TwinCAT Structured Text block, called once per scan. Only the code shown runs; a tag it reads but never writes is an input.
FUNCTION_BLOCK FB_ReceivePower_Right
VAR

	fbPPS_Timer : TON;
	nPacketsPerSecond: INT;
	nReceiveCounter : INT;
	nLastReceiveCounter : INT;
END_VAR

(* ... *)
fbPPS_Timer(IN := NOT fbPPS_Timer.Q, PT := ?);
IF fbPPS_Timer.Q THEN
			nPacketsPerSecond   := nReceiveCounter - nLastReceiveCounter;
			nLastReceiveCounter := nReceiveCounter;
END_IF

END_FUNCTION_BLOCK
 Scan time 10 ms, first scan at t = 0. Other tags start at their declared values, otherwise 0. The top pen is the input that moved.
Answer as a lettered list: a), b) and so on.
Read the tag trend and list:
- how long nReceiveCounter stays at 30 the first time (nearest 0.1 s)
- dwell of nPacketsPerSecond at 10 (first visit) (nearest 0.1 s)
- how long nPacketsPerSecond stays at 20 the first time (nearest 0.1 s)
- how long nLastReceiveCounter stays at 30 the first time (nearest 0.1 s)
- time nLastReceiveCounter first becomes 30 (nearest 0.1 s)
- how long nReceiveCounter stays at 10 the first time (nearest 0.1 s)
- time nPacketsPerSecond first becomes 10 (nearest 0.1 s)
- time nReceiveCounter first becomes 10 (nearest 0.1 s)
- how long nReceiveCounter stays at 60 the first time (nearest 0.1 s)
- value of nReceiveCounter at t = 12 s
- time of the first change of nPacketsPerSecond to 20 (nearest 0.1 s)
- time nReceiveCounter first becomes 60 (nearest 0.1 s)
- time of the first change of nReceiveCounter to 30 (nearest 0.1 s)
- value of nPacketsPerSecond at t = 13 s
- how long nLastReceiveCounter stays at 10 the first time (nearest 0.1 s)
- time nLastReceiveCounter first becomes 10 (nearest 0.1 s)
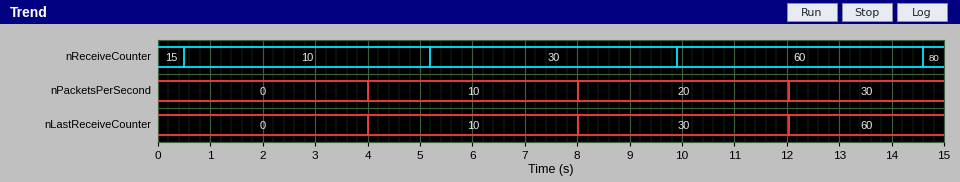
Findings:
a) 4.7 s
b) 4.0 s
c) 4.0 s
d) 4.0 s
e) 8.0 s
f) 4.7 s
g) 4.0 s
h) 0.5 s
i) 4.7 s
j) 60
k) 8.0 s
l) 9.9 s
m) 5.2 s
n) 30
o) 4.0 s
p) 4.0 s
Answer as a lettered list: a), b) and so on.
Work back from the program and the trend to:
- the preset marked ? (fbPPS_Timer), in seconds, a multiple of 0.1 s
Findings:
a) 4.0 s
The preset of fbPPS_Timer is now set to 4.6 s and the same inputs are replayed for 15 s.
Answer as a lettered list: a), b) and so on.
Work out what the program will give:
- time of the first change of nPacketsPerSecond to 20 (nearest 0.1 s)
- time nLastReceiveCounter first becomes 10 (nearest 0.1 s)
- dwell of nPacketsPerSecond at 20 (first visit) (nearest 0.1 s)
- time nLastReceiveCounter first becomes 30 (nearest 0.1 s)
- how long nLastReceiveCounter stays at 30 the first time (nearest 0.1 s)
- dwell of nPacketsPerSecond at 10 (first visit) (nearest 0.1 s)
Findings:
a) 9.2 s
b) 4.6 s
c) 4.6 s
d) 9.2 s
e) 4.6 s
f) 4.6 s
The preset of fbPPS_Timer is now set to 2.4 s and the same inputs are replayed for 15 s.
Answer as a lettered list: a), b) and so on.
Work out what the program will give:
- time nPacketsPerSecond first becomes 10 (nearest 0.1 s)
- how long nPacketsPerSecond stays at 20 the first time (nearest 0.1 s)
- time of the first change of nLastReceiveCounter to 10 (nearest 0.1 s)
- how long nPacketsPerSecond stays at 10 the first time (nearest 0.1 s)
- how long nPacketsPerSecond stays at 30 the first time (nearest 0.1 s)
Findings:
a) 2.4 s
b) 2.4 s
c) 2.4 s
d) 2.4 s
e) 2.4 s
